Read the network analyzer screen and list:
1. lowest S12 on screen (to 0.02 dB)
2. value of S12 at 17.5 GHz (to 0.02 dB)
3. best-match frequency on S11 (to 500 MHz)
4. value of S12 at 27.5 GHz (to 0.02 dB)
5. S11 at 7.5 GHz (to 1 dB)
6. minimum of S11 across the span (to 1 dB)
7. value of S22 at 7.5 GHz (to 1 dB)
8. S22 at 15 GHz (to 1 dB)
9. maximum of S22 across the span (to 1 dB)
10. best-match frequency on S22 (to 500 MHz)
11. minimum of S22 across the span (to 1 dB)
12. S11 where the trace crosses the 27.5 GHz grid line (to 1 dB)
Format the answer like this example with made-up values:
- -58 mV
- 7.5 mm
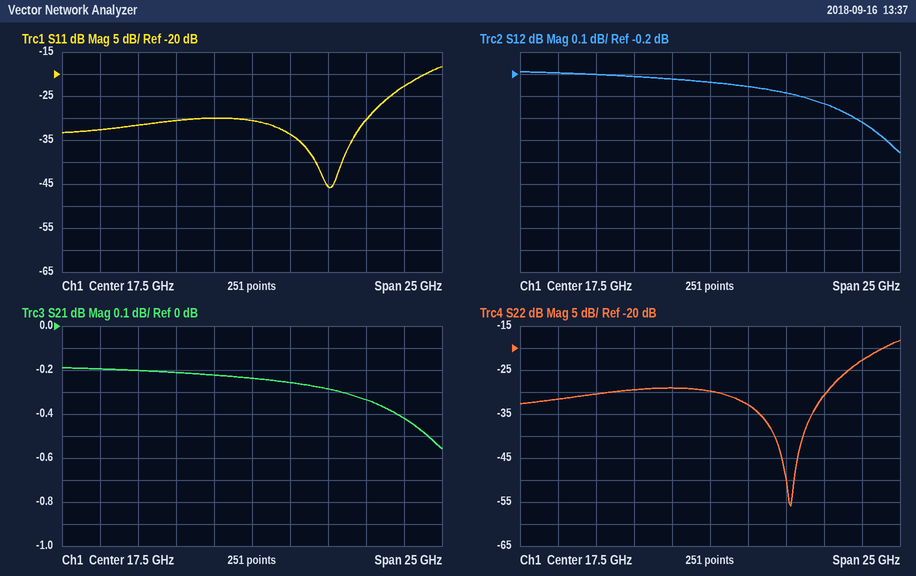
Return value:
- -0.56 dB
- -0.24 dB
- 22.5 GHz
- -0.42 dB
- -33 dB
- -46 dB
- -32 dB
- -29 dB
- -18 dB
- 23.0 GHz
- -56 dB
- -23 dB
